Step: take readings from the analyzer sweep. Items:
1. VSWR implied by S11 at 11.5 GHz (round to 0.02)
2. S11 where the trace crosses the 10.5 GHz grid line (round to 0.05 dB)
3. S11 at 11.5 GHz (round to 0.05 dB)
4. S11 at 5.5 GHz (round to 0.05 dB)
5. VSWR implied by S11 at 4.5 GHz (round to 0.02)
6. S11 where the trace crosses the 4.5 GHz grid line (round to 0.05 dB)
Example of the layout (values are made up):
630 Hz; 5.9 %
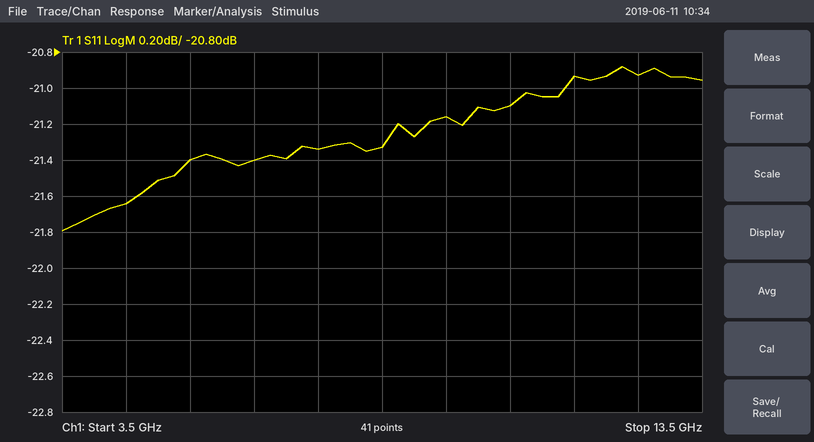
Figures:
1.20; -21.10 dB; -20.95 dB; -21.40 dB; 1.18; -21.65 dB
